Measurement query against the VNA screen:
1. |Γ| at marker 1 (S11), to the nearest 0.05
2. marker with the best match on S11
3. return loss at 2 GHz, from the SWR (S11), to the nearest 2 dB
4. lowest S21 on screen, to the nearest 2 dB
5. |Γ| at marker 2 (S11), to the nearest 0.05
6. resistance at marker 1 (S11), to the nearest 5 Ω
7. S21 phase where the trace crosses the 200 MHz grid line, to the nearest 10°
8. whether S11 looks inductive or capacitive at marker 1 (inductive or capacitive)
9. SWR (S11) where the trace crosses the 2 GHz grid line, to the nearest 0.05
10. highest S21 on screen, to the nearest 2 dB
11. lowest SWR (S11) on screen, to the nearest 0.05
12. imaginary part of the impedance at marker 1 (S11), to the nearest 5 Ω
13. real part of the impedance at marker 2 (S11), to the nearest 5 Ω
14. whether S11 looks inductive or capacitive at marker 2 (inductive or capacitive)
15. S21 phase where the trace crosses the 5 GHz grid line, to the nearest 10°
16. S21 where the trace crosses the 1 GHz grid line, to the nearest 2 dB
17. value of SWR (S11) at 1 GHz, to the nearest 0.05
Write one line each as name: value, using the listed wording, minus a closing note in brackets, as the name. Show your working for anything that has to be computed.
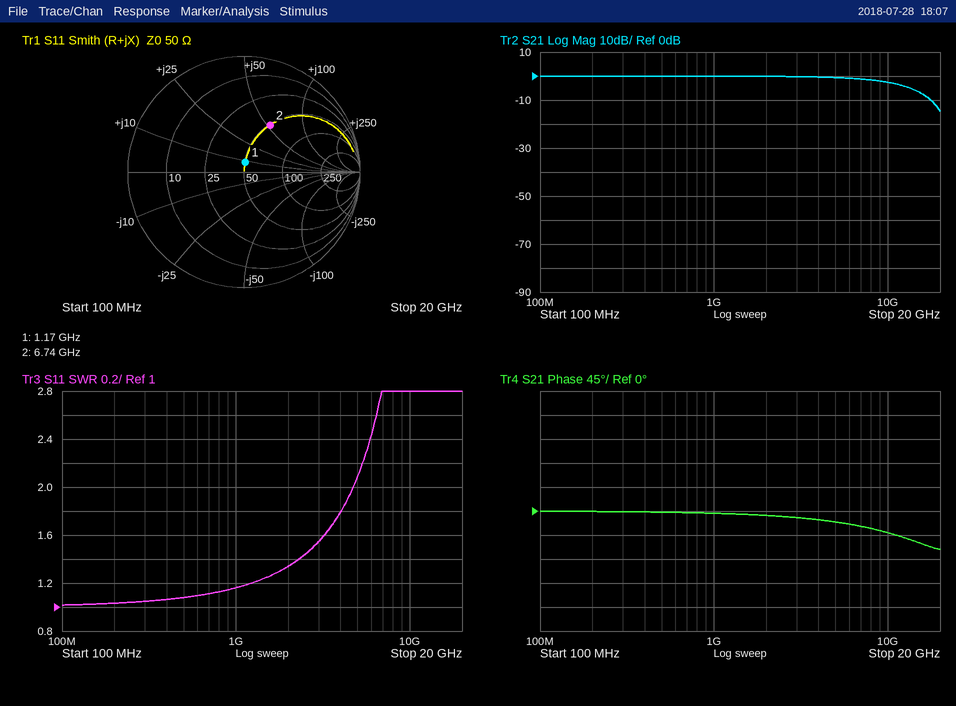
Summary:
|Γ| at marker 1 (S11), to the nearest 0.05: 0.10
marker with the best match on S11: marker 1
return loss at 2 GHz, from the SWR (S11), to the nearest 2 dB: −20 log10((1.35 − 1)/(1.35 + 1)) ≈ 16 dB
lowest S21 on screen, to the nearest 2 dB: -14 dB
|Γ| at marker 2 (S11), to the nearest 0.05: 0.45
resistance at marker 1 (S11), to the nearest 5 Ω: 50 Ω
S21 phase where the trace crosses the 200 MHz grid line, to the nearest 10°: 0°
whether S11 looks inductive or capacitive at marker 1: inductive
SWR (S11) where the trace crosses the 2 GHz grid line, to the nearest 0.05: 1.35
highest S21 on screen, to the nearest 2 dB: 0 dB
lowest SWR (S11) on screen, to the nearest 0.05: 1.00
imaginary part of the impedance at marker 1 (S11), to the nearest 5 Ω: +10 Ω
real part of the impedance at marker 2 (S11), to the nearest 5 Ω: 50 Ω
whether S11 looks inductive or capacitive at marker 2: inductive
S21 phase where the trace crosses the 5 GHz grid line, to the nearest 10°: -20°
S21 where the trace crosses the 1 GHz grid line, to the nearest 2 dB: 0 dB
value of SWR (S11) at 1 GHz, to the nearest 0.05: 1.15
